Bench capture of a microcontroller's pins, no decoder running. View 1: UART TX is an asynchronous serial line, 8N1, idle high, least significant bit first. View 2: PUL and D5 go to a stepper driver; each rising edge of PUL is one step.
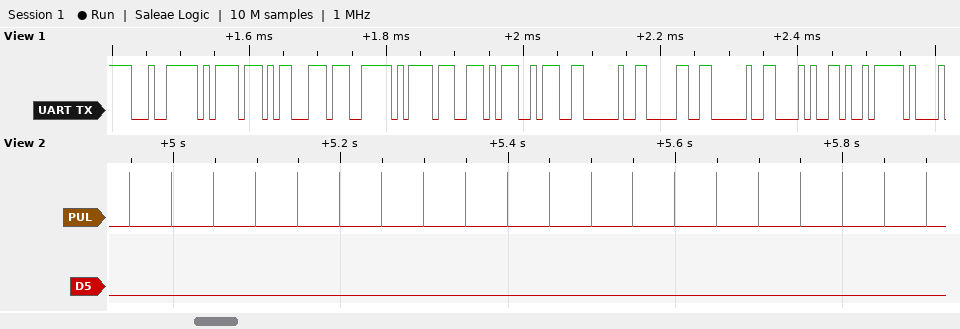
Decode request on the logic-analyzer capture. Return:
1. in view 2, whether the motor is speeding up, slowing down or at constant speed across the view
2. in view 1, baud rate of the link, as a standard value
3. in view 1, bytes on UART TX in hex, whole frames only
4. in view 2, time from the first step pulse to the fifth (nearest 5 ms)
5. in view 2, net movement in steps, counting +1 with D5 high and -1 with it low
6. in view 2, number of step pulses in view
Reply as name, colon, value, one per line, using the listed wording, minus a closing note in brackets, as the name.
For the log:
in view 2, whether the motor is speeding up, slowing down or at constant speed across the view: constant speed
in view 1, baud rate of the link, as a standard value: 115200 baud
in view 1, bytes on UART TX in hex, whole frames only: E4 BD 8D E7 BD AE 3A 20 30 20 28 E9
in view 2, time from the first step pulse to the fifth: 200 ms
in view 2, net movement in steps, counting +1 with D5 high and -1 with it low: -20
in view 2, number of step pulses in view: 20
